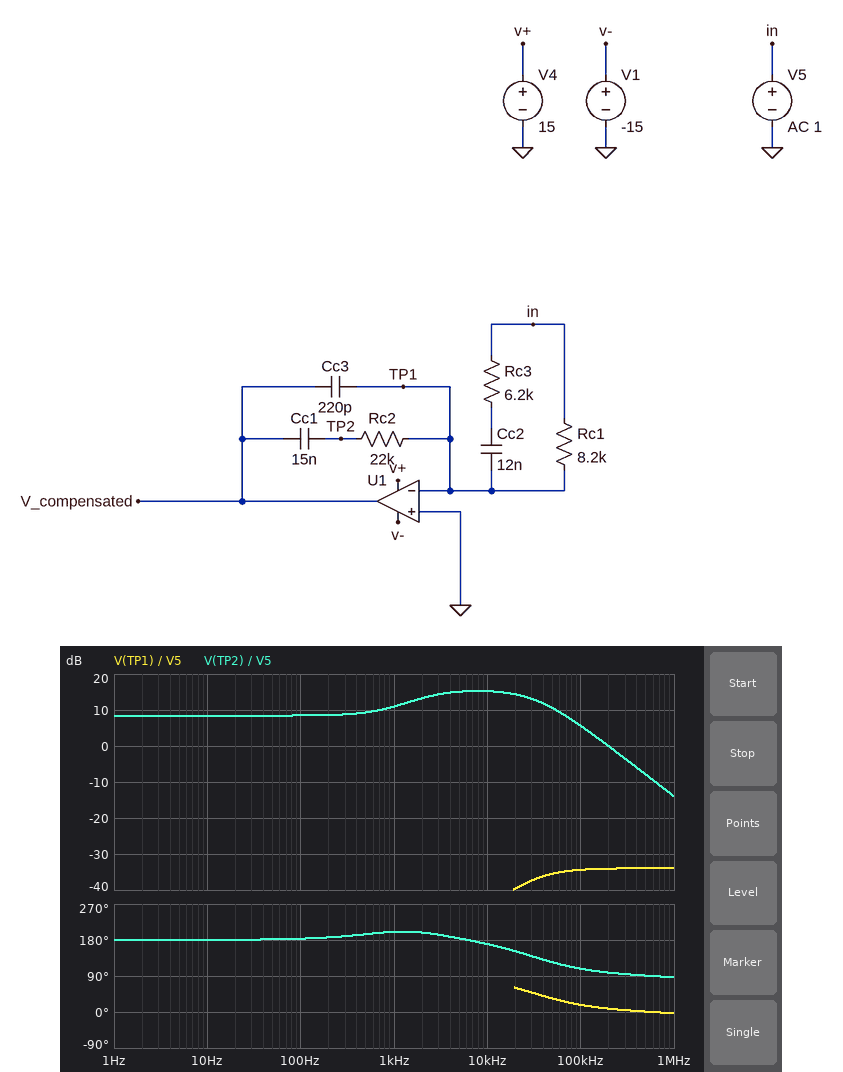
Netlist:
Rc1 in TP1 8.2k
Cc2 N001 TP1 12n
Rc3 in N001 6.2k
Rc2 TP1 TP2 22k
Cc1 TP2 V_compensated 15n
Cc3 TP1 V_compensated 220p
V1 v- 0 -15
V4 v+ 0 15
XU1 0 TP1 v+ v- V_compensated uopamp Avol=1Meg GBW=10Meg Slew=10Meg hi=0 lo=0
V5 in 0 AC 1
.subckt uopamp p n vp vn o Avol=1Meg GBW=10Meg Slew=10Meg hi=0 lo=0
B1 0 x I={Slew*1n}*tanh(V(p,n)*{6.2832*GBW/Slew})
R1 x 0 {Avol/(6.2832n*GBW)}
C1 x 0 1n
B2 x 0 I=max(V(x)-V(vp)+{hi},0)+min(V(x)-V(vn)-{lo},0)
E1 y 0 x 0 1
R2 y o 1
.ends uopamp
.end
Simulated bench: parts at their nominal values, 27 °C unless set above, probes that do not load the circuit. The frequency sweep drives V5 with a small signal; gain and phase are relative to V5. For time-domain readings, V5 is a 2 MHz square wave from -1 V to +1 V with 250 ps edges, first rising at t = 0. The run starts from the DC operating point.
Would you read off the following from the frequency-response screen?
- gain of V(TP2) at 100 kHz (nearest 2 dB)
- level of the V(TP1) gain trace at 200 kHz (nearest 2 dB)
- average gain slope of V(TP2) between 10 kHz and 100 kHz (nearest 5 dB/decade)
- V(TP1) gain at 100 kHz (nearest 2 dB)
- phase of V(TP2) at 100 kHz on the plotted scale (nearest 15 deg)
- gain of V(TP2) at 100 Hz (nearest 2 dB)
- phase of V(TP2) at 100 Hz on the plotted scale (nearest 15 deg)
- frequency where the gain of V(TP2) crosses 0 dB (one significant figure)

6 dB
-34 dB
-10 dB/decade
-34 dB
105 deg
8 dB
180 deg
200 kHz
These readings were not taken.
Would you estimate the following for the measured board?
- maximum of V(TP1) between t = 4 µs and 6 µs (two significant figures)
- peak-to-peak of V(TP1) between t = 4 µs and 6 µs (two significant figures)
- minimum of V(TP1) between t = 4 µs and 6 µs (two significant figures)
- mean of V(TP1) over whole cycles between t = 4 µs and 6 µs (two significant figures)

6.0 mV
310 mV
-300 mV
-150 mV
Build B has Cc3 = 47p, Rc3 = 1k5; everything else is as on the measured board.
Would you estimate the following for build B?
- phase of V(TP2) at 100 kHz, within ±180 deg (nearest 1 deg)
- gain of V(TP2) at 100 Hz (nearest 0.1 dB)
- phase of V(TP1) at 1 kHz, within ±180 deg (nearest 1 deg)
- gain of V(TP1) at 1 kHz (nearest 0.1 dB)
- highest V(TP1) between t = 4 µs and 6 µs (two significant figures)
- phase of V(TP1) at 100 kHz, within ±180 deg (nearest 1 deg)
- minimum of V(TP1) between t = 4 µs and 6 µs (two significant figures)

144 deg
8.6 dB
93 deg
-68.7 dB
280 mV
54 deg
-730 mV
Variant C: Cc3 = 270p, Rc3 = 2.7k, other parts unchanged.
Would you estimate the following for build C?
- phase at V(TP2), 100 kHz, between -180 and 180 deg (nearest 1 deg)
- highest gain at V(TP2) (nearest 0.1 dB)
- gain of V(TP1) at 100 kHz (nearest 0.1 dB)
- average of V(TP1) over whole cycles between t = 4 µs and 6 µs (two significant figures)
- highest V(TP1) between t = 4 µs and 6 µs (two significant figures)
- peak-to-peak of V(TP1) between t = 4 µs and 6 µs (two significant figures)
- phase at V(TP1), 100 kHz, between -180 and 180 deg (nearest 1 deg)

106 deg
19.1 dB
-31.3 dB
-100 mV
25 mV
330 mV
16 deg
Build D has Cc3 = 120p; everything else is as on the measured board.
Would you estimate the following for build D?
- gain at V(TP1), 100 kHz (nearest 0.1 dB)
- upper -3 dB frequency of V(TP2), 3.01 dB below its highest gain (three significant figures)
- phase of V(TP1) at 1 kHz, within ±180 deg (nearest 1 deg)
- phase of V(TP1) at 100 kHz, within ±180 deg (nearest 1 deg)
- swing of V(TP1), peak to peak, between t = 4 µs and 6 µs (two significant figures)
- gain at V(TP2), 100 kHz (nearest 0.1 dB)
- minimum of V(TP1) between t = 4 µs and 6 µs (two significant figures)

-30.1 dB
62.3 kHz
85 deg
30 deg
440 mV
9.9 dB
-410 mV
